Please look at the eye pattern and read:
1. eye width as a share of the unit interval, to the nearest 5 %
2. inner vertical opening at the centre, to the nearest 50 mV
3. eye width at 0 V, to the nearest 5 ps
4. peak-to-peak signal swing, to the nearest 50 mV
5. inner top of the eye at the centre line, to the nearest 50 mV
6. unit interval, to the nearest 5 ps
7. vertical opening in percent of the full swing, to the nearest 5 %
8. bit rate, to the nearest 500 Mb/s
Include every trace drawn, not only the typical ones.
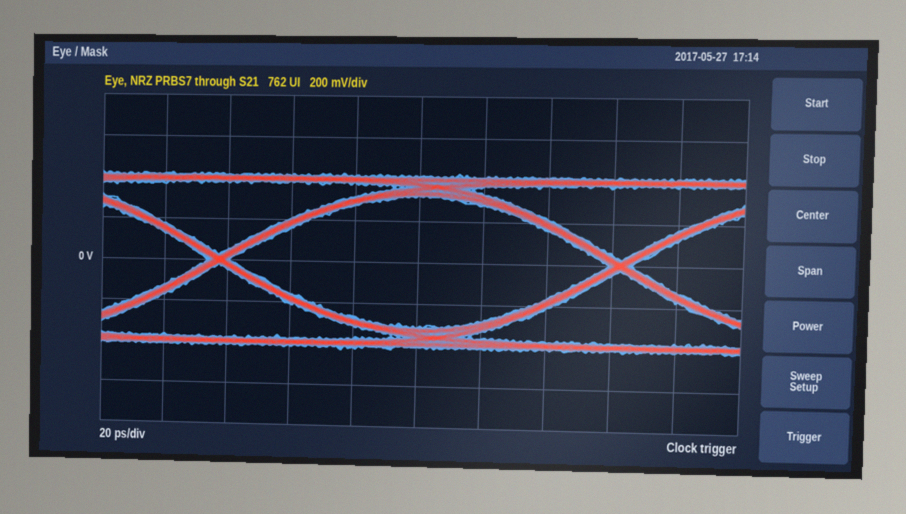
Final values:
95 %
650 mV
120 ps
850 mV
300 mV
125 ps
75 %
8.0 Gb/s
